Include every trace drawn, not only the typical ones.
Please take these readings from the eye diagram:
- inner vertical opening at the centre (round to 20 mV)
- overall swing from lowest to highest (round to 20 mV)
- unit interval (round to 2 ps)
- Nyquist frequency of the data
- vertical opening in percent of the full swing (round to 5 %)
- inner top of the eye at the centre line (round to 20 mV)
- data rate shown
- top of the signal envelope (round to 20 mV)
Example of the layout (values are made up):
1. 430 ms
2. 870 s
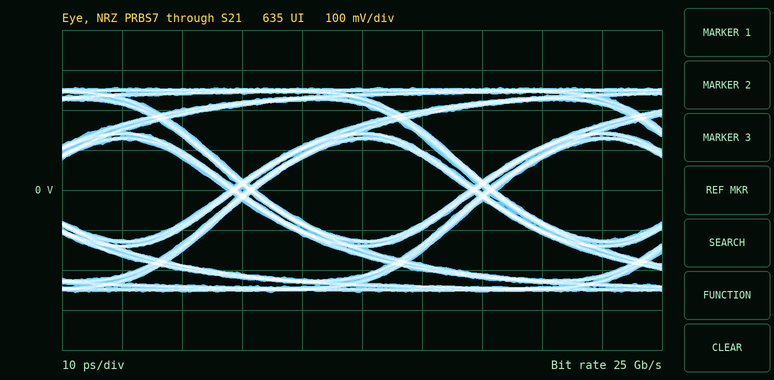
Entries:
1. 260 mV
2. 520 mV
3. 40 ps
4. 12.5 GHz
5. 50 %
6. 120 mV
7. 25 Gb/s
8. 260 mV
